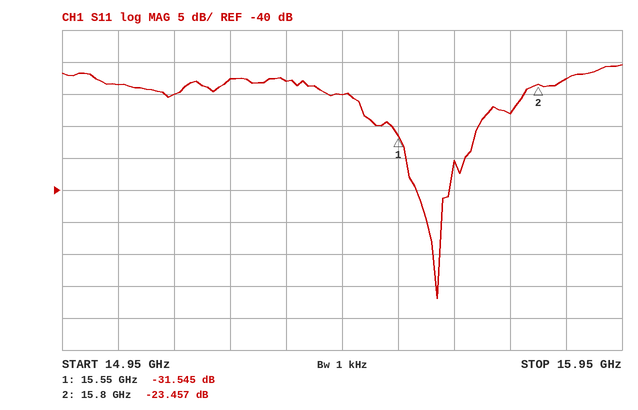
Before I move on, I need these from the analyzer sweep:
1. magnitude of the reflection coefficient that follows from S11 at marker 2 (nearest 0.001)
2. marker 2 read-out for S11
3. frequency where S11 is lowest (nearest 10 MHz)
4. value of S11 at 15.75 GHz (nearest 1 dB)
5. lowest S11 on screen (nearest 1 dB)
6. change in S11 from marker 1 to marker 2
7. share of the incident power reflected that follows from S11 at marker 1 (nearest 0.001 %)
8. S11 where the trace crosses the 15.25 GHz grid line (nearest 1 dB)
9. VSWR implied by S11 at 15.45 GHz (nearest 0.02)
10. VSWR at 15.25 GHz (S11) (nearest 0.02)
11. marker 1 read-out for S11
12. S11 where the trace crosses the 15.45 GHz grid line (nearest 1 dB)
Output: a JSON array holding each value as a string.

["0.067", "-23.457 dB", "15.62 GHz", "-28 dB", "-57 dB", "8.088 dB", "0.070 %", "-23 dB", "1.12", "1.16", "-31.545 dB", "-25 dB"]
